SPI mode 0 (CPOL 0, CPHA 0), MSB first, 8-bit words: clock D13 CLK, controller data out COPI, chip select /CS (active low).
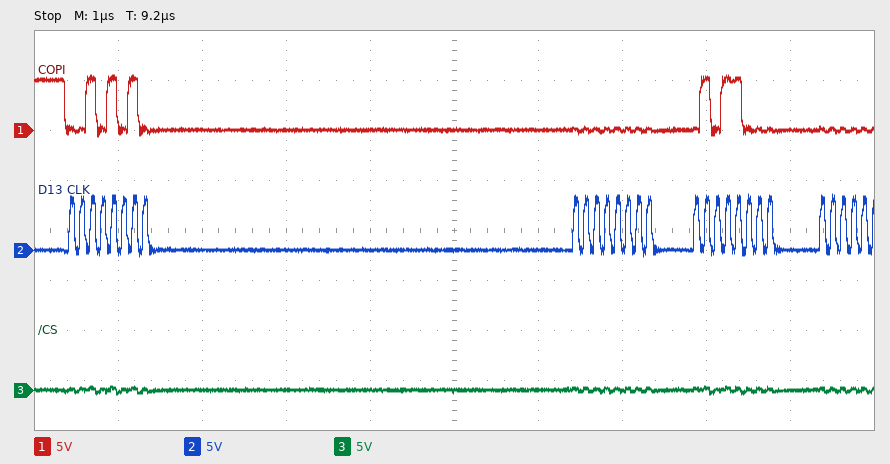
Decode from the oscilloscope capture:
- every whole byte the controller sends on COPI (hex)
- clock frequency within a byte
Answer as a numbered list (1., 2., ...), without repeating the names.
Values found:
1. 0x2A 0x00 0x58
2. 8 MHz
